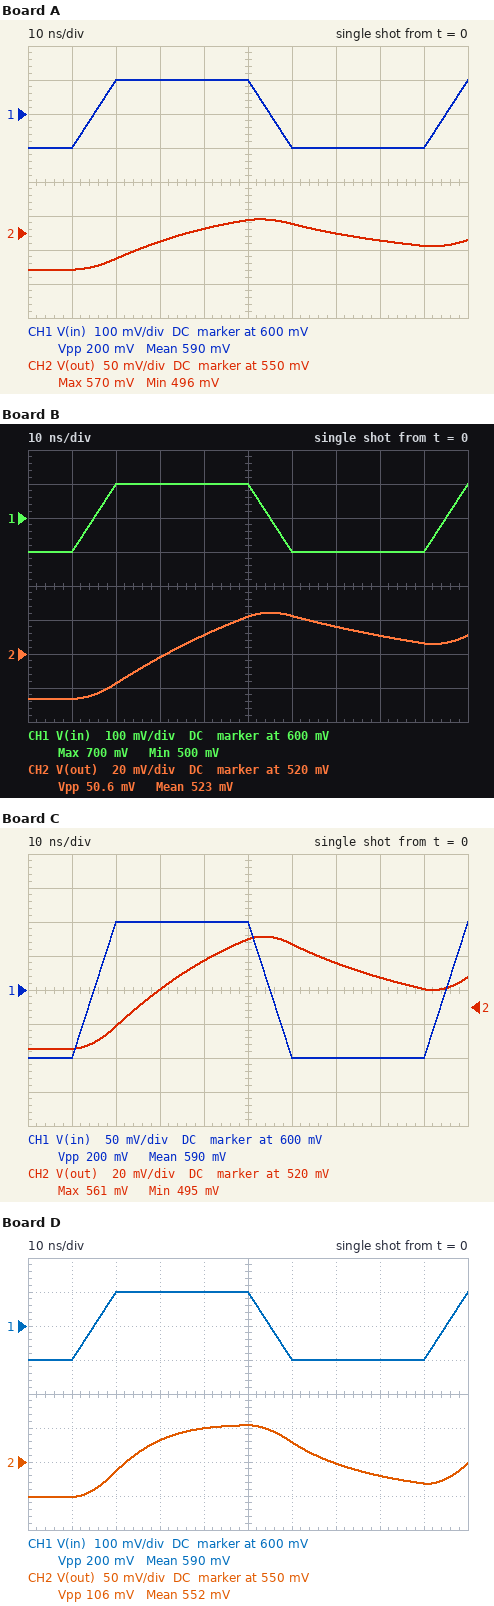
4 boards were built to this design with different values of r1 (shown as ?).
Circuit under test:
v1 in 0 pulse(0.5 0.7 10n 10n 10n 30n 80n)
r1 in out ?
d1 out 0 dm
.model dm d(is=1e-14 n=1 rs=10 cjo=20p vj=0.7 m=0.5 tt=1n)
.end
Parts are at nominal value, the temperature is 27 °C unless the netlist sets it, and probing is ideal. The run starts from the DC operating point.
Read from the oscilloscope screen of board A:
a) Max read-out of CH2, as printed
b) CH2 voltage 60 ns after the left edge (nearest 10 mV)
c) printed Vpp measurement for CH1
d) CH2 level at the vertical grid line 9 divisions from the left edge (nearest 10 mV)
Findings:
570 mV
560 mV
200 mV
530 mV
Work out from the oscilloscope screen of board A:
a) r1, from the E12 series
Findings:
1.8 kΩ
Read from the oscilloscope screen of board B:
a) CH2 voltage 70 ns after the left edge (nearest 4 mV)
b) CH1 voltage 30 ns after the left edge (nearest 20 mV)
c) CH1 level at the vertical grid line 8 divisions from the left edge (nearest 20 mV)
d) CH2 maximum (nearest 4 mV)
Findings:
536 mV
700 mV
500 mV
544 mV
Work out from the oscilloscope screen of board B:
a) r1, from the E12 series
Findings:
3.3 kΩ
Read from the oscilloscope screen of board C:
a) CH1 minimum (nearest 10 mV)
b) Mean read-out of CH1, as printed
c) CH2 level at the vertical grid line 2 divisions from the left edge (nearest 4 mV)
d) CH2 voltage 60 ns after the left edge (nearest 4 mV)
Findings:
500 mV
590 mV
508 mV
556 mV
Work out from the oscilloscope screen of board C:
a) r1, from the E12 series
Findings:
2.2 kΩ
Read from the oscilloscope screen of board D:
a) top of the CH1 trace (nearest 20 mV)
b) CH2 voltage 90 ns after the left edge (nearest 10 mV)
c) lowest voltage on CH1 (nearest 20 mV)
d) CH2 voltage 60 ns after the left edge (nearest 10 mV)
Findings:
700 mV
520 mV
500 mV
580 mV
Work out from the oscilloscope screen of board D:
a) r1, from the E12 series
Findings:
680 Ω
